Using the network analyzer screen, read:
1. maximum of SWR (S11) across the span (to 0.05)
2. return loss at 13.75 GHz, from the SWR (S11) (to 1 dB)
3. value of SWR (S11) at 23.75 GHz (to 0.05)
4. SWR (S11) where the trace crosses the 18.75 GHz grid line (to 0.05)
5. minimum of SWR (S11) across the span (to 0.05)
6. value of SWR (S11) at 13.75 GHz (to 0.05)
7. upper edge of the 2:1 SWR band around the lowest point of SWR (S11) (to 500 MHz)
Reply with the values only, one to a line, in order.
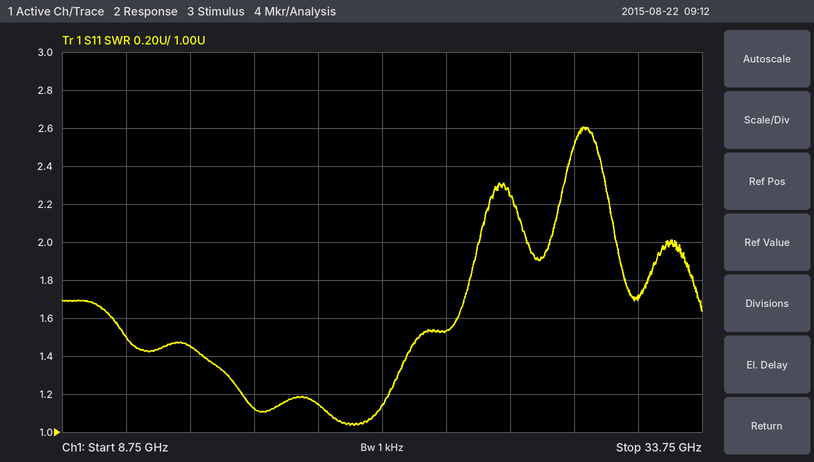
2.60
15 dB
1.55
1.15
1.05
1.45
25.0 GHz
